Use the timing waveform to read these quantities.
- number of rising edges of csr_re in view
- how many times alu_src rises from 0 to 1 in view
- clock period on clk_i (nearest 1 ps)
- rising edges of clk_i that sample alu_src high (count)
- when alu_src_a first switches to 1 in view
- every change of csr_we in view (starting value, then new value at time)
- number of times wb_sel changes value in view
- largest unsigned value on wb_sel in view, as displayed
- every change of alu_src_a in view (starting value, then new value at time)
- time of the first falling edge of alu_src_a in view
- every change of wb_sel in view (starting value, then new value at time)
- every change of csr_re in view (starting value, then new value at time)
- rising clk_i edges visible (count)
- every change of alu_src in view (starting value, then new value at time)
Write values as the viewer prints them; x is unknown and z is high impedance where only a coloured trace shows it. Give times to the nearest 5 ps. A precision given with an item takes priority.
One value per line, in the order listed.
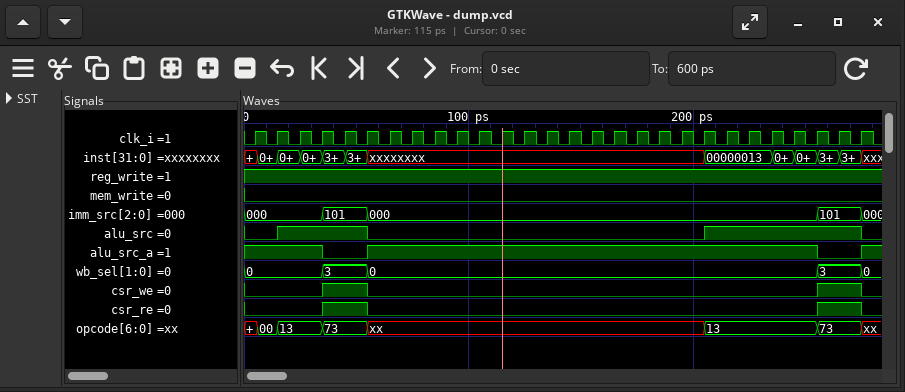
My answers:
2
2
10 ps
11
55 ps
0, 1 at 35 ps, 0 at 55 ps, 1 at 255 ps, 0 at 275 ps
4
3
1, 0 at 35 ps, 1 at 55 ps, 0 at 255 ps, 1 at 275 ps
35 ps
0, 3 at 35 ps, 0 at 55 ps, 3 at 255 ps, 0 at 275 ps
0, 1 at 35 ps, 0 at 55 ps, 1 at 255 ps, 0 at 275 ps
28
0, 1 at 15 ps, 0 at 55 ps, 1 at 205 ps, 0 at 275 ps
